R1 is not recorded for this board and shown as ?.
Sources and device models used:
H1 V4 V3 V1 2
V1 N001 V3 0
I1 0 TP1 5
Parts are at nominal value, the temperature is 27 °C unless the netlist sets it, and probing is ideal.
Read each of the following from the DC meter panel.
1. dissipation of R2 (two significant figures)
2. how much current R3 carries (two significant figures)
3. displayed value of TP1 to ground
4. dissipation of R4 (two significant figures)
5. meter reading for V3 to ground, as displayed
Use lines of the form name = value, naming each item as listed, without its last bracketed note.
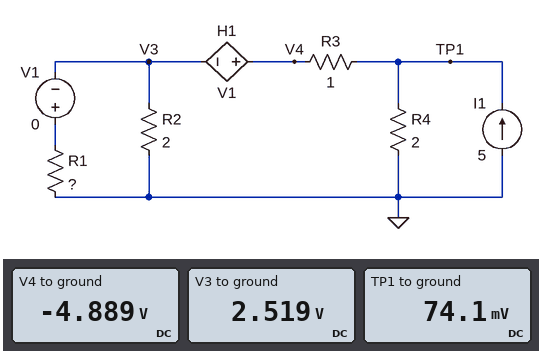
dissipation of R2 = 3.2 W
how much current R3 carries = 5.0 A
displayed value of TP1 to ground = 74.1 mV
dissipation of R4 = 2.7 mW
meter reading for V3 to ground, as displayed = 2.519 V
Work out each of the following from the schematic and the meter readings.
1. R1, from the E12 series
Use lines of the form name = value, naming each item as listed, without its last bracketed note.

R1, from the E12 series = 0.68 Ω
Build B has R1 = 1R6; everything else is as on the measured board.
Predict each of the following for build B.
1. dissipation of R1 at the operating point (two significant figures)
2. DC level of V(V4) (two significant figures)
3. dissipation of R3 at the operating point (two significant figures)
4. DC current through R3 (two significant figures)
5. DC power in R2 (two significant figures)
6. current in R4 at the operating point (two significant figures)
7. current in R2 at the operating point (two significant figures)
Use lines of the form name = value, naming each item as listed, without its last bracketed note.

dissipation of R1 at the operating point = 6.4 W
DC level of V(V4) = -800 mV
dissipation of R3 at the operating point = 13 W
DC current through R3 = 3.6 A
DC power in R2 = 5.1 W
current in R4 at the operating point = 1.4 A
current in R2 at the operating point = 1.6 A
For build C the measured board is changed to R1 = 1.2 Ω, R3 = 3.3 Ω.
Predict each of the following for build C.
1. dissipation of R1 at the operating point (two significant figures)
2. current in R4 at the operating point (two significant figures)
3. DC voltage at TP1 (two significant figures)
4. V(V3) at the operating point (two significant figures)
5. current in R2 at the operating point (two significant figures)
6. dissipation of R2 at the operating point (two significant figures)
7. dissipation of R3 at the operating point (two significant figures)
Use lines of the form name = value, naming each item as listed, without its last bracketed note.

dissipation of R1 at the operating point = 2.0 W
current in R4 at the operating point = 2.9 A
DC voltage at TP1 = 5.8 V
V(V3) at the operating point = 1.6 V
current in R2 at the operating point = 780 mA
dissipation of R2 at the operating point = 1.2 W
dissipation of R3 at the operating point = 14 W
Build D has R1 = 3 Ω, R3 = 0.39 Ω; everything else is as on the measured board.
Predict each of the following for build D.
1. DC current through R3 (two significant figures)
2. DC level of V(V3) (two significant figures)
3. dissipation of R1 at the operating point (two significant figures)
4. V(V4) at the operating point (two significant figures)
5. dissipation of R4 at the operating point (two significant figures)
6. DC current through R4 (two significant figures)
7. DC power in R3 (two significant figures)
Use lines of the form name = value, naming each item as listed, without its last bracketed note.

DC current through R3 = 3.6 A
DC level of V(V3) = 4.3 V
dissipation of R1 at the operating point = 6.2 W
V(V4) at the operating point = 1.4 V
dissipation of R4 at the operating point = 4.0 W
DC current through R4 = 1.4 A
DC power in R3 = 5.0 W
